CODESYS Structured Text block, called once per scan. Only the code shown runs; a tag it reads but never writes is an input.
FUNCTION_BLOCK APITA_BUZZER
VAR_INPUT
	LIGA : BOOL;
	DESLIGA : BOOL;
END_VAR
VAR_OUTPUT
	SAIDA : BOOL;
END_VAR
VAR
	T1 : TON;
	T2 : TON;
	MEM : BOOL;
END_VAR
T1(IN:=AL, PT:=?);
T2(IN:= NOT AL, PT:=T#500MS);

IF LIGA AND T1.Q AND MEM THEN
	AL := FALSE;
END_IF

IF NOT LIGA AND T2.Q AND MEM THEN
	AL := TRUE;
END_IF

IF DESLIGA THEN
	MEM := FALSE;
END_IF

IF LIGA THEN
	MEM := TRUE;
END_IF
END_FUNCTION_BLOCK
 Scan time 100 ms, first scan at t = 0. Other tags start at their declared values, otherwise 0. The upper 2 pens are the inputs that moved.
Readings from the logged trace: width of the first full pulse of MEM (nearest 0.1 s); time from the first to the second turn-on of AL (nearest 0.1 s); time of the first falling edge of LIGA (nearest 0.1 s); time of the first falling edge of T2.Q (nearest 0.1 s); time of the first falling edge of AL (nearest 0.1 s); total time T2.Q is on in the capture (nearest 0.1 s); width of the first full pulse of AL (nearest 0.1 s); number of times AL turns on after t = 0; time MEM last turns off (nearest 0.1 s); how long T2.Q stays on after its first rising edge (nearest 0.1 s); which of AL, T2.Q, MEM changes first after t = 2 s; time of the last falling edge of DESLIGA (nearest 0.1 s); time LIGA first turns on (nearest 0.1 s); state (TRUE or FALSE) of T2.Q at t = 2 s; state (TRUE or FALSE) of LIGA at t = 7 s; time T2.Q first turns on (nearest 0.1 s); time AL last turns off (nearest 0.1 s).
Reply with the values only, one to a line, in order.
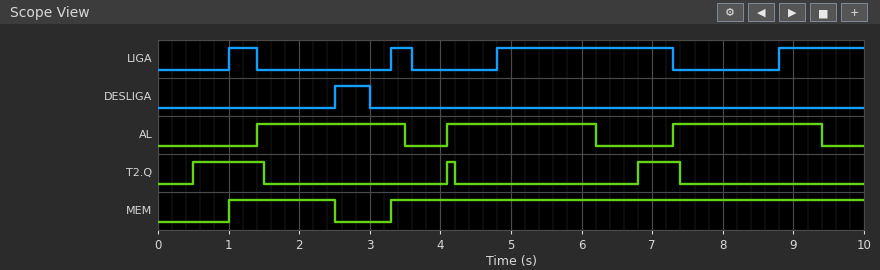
1.5 s
2.7 s
1.4 s
1.5 s
3.5 s
1.7 s
2.1 s
3
2.5 s
1.0 s
MEM
3.0 s
1.0 s
FALSE
TRUE
0.5 s
9.4 s
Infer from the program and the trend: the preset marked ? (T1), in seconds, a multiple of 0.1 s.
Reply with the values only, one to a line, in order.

2.0 s
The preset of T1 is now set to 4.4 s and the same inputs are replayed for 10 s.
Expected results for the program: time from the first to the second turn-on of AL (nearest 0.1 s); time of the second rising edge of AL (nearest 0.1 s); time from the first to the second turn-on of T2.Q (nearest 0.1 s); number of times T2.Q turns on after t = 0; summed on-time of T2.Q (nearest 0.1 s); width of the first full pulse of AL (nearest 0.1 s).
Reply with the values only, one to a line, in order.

5.9 s
7.3 s
6.0 s
2
1.9 s
4.5 s
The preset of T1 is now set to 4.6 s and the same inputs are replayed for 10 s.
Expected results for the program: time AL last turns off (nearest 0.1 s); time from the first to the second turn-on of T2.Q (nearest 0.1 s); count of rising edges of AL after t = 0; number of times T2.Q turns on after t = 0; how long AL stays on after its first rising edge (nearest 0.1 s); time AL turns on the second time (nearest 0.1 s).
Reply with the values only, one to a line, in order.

6.1 s
6.2 s
2
2
4.7 s
7.3 s
